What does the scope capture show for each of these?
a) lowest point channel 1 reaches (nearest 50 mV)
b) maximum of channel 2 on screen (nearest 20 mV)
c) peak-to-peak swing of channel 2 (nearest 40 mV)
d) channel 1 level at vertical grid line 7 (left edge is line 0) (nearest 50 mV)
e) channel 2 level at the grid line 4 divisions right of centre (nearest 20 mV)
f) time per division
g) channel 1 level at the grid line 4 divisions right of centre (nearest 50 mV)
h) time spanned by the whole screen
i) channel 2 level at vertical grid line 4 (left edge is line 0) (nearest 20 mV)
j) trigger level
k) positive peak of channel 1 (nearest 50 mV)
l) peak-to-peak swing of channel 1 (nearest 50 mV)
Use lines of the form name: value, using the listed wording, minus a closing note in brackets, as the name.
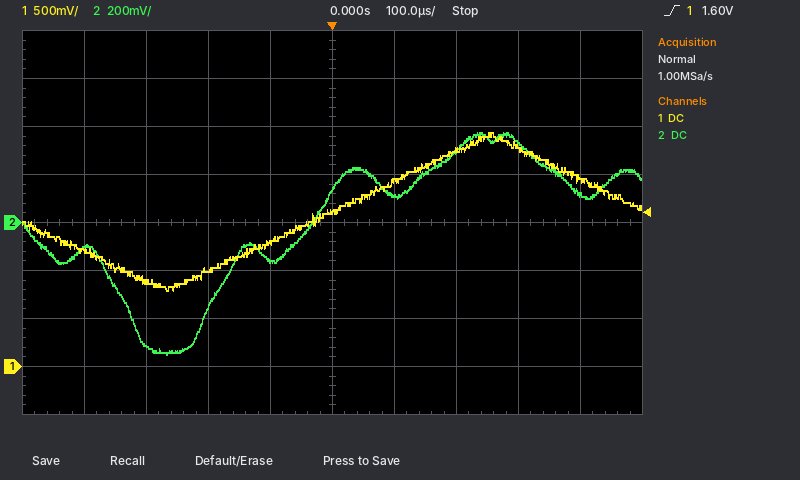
lowest point channel 1 reaches: 800 mV
maximum of channel 2 on screen: 380 mV
peak-to-peak swing of channel 2: 920 mV
channel 1 level at vertical grid line 7 (left edge is line 0): 2.25 V
channel 2 level at the grid line 4 divisions right of centre: 120 mV
time per division: 100 µs
channel 1 level at the grid line 4 divisions right of centre: 1.95 V
time spanned by the whole screen: 1 ms
channel 2 level at vertical grid line 4 (left edge is line 0): -160 mV
trigger level: 1.60 V
positive peak of channel 1: 2.45 V
peak-to-peak swing of channel 1: 1.65 V
